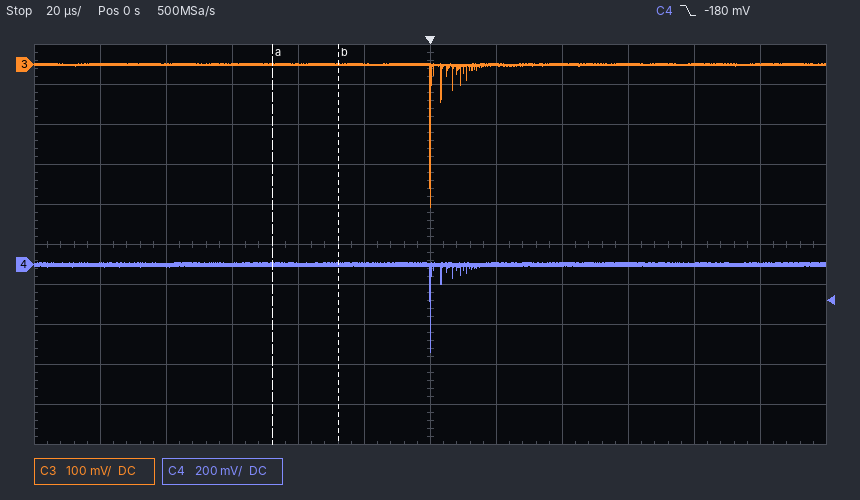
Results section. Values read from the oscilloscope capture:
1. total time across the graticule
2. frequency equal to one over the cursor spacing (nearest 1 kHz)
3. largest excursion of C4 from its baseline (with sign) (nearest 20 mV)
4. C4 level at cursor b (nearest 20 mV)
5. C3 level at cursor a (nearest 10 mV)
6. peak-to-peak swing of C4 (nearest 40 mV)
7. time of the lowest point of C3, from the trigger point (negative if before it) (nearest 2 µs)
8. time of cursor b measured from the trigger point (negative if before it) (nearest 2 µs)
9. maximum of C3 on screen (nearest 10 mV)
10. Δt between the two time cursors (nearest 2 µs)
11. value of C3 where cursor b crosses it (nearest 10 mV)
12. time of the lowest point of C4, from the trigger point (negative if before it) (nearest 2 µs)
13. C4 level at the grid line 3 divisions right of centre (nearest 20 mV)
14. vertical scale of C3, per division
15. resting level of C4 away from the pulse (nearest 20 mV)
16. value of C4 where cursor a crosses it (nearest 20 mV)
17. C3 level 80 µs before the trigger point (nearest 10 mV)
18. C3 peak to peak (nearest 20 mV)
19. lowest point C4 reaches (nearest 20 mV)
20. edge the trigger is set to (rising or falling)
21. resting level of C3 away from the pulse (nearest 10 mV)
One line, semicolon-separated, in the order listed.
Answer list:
240 µs; 50 kHz; -440 mV; 0 mV; 0 mV; 440 mV; 0 µs; -28 µs; 0 mV; 20 µs; 0 mV; 0 µs; 0 mV; 100 mV; 0 mV; 0 mV; 0 mV; 360 mV; -440 mV; falling; 0 mV
